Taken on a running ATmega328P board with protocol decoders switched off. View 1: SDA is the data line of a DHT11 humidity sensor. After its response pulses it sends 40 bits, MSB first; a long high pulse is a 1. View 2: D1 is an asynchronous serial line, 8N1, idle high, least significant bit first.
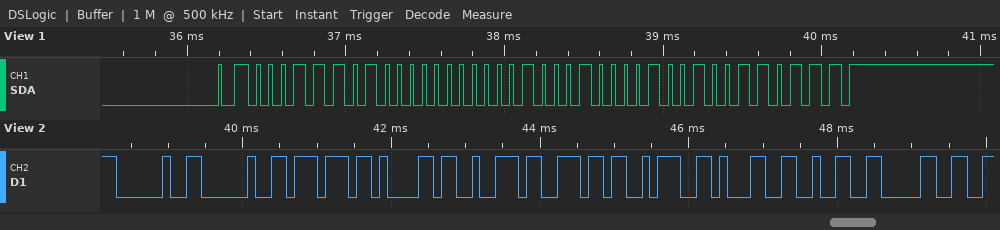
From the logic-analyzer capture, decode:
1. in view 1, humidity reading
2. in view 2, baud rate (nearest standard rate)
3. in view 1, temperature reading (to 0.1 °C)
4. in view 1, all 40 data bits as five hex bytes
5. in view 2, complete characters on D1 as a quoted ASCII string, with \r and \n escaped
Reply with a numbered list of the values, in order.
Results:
1. 29 %
2. 9600 baud
3. 17.9 °C
4. 1D 00 11 09 37
5. "  warn:120"
